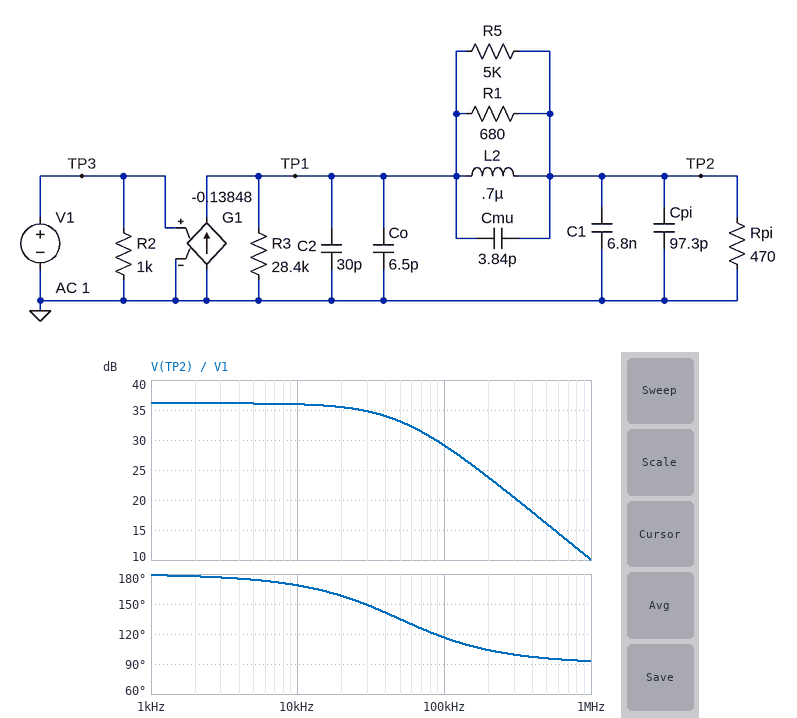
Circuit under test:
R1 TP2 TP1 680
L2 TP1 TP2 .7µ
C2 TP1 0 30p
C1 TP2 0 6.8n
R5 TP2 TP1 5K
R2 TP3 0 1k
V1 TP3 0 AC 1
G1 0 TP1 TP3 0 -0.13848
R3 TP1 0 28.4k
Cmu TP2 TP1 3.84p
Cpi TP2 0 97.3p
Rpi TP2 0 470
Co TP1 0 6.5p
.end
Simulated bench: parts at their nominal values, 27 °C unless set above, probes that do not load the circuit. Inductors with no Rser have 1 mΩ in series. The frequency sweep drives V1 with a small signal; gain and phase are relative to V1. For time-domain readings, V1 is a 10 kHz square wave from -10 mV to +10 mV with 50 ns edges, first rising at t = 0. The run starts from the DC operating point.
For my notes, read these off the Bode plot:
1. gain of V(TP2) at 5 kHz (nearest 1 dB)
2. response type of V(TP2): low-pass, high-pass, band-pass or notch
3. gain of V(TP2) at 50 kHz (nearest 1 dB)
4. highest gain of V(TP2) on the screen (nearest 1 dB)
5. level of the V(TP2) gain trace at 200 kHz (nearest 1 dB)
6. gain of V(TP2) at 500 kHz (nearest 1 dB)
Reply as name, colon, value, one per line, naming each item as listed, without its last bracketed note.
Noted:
gain of V(TP2) at 5 kHz: 36 dB
response type of V(TP2): low-pass, high-pass, band-pass or notch: low-pass
gain of V(TP2) at 50 kHz: 33 dB
highest gain of V(TP2) on the screen: 36 dB
level of the V(TP2) gain trace at 200 kHz: 24 dB
gain of V(TP2) at 500 kHz: 16 dB
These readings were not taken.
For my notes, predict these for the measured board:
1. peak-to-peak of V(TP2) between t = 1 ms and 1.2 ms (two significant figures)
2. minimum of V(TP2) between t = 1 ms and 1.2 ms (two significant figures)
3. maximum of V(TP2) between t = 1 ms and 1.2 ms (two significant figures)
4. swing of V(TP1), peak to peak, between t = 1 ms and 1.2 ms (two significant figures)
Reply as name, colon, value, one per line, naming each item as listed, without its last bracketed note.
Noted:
peak-to-peak of V(TP2) between t = 1 ms and 1.2 ms: 1.3 V
minimum of V(TP2) between t = 1 ms and 1.2 ms: -640 mV
maximum of V(TP2) between t = 1 ms and 1.2 ms: 640 mV
swing of V(TP1), peak to peak, between t = 1 ms and 1.2 ms: 1.3 V
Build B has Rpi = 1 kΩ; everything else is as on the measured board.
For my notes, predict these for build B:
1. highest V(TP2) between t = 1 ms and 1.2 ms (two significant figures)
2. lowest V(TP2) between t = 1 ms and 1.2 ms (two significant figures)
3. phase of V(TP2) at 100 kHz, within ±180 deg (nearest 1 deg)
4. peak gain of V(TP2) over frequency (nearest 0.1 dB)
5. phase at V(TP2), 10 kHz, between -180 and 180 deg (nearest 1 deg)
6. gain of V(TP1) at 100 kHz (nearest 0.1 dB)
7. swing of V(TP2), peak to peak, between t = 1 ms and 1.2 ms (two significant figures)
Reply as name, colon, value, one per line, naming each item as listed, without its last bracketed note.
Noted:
highest V(TP2) between t = 1 ms and 1.2 ms: 1.3 V
lowest V(TP2) between t = 1 ms and 1.2 ms: -1.3 V
phase of V(TP2) at 100 kHz, within ±180 deg: 103 deg
peak gain of V(TP2) over frequency: 42.5 dB
phase at V(TP2), 10 kHz, between -180 and 180 deg: 157 deg
gain of V(TP1) at 100 kHz: 29.8 dB
swing of V(TP2), peak to peak, between t = 1 ms and 1.2 ms: 2.7 V
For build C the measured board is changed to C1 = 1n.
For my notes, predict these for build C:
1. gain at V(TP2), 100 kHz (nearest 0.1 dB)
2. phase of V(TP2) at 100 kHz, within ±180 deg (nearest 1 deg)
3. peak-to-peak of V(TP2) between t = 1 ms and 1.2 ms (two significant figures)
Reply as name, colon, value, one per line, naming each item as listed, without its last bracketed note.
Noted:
gain at V(TP2), 100 kHz: 35.7 dB
phase of V(TP2) at 100 kHz, within ±180 deg: 162 deg
peak-to-peak of V(TP2) between t = 1 ms and 1.2 ms: 1.3 V
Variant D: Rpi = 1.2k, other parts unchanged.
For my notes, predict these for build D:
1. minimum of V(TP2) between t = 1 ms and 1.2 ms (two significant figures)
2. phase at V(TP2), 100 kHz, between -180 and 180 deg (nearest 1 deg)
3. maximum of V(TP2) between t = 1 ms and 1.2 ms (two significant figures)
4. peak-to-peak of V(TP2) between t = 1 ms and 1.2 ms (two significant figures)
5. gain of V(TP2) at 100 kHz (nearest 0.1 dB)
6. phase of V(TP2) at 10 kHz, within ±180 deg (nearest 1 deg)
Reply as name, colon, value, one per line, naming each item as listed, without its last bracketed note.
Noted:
minimum of V(TP2) between t = 1 ms and 1.2 ms: -1.6 V
phase at V(TP2), 100 kHz, between -180 and 180 deg: 101 deg
maximum of V(TP2) between t = 1 ms and 1.2 ms: 1.6 V
peak-to-peak of V(TP2) between t = 1 ms and 1.2 ms: 3.2 V
gain of V(TP2) at 100 kHz: 29.9 dB
phase of V(TP2) at 10 kHz, within ±180 deg: 153 deg
